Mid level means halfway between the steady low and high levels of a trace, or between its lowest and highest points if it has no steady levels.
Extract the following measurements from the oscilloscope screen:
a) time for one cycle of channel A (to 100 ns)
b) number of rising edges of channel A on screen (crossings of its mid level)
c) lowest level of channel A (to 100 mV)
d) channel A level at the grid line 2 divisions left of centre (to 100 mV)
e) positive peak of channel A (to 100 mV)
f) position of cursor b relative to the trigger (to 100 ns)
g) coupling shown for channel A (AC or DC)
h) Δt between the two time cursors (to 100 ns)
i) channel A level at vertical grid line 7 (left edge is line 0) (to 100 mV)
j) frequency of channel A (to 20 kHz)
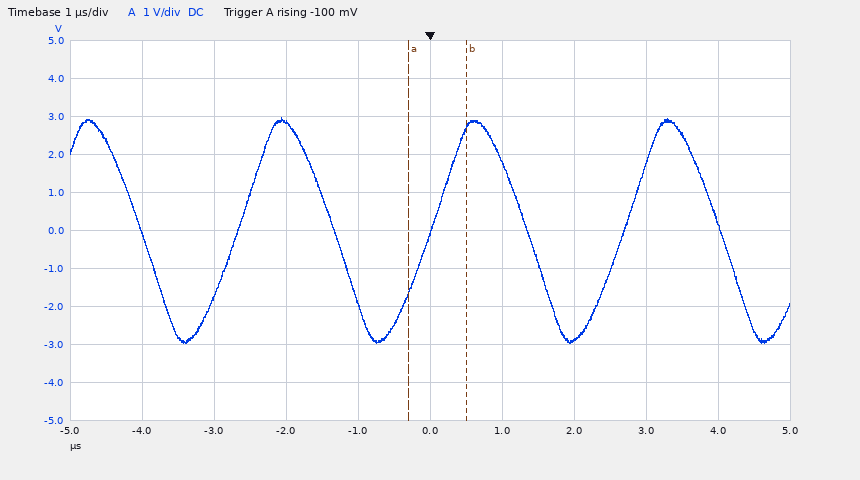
2.7 µs
3
-3.0 V
2.8 V
3.0 V
+500 ns
DC
800 ns
-2.9 V
380 kHz
